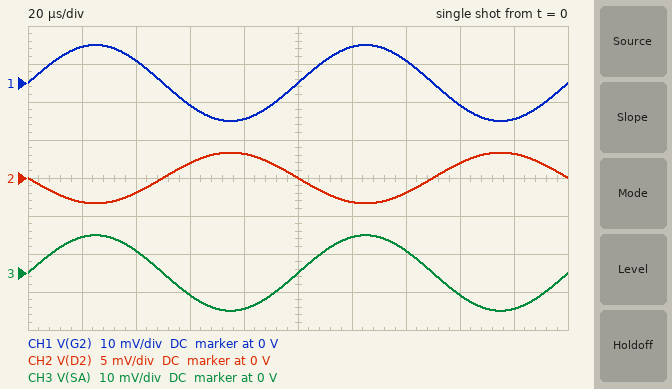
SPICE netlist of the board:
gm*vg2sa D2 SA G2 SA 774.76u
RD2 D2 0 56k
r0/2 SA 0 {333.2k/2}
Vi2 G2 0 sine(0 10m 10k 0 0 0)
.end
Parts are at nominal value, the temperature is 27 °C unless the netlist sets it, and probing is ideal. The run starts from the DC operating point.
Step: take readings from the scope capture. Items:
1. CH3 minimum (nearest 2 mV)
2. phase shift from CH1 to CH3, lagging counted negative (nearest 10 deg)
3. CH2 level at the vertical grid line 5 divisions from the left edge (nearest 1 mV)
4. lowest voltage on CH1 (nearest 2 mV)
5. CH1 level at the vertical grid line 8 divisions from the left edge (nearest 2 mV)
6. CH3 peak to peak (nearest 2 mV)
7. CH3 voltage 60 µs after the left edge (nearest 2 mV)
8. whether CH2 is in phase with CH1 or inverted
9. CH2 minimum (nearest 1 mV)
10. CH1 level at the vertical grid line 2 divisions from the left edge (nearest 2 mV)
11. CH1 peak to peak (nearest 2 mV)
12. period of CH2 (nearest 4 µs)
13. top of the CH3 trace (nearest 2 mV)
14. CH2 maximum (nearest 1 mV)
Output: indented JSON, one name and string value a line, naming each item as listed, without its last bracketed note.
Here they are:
{
  "CH3 minimum": "-10 mV",
  "phase shift from CH1 to CH3, lagging counted negative": "0 deg",
  "CH2 level at the vertical grid line 5 divisions from the left edge": "0 V",
  "lowest voltage on CH1": "-10 mV",
  "CH1 level at the vertical grid line 8 divisions from the left edge": "-6 mV",
  "CH3 peak to peak": "20 mV",
  "CH3 voltage 60 µs after the left edge": "-6 mV",
  "whether CH2 is in phase with CH1 or inverted": "inverted",
  "CH2 minimum": "-3 mV",
  "CH1 level at the vertical grid line 2 divisions from the left edge": "6 mV",
  "CH1 peak to peak": "20 mV",
  "period of CH2": "100 µs",
  "top of the CH3 trace": "10 mV",
  "CH2 maximum": "3 mV"
}
